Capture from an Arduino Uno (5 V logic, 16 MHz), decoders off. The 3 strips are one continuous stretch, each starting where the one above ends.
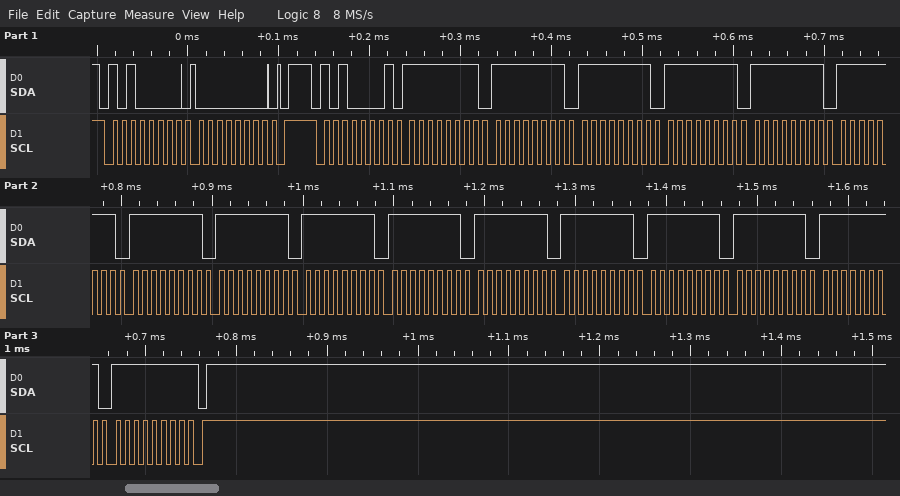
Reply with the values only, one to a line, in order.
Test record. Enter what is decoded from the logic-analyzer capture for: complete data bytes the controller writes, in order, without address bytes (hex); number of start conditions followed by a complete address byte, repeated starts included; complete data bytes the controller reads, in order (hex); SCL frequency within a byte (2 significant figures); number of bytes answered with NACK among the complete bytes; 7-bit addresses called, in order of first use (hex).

00
2
FF FF FF FF FF FF FF FF FF FF FF FF FF FF FF FF
100 kHz
1
0x50
